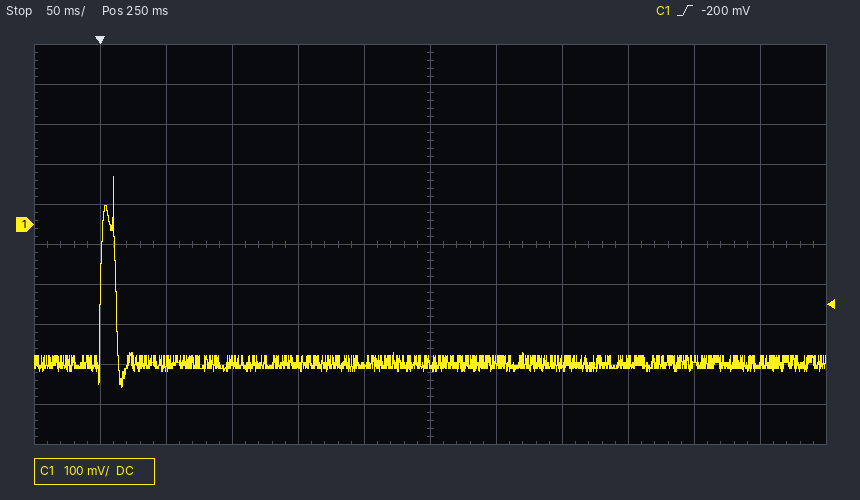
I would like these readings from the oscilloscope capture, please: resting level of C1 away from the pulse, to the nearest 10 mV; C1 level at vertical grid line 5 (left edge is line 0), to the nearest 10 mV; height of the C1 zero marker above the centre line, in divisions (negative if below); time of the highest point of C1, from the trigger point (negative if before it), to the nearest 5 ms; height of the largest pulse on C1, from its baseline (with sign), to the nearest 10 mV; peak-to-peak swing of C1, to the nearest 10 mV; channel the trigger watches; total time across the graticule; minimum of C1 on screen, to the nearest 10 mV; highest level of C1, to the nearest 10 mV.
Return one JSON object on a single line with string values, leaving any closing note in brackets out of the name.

{"resting level of C1 away from the pulse, to the nearest 10 mV": "-340 mV", "C1 level at vertical grid line 5 (left edge is line 0), to the nearest 10 mV": "-350 mV", "height of the C1 zero marker above the centre line, in divisions": "+0.5 div", "time of the highest point of C1, from the trigger point (negative if before it), to the nearest 5 ms": "+10 ms", "height of the largest pulse on C1, from its baseline (with sign), to the nearest 10 mV": "+460 mV", "peak-to-peak swing of C1, to the nearest 10 mV": "530 mV", "channel the trigger watches": "C1", "total time across the graticule": "600 ms", "minimum of C1 on screen, to the nearest 10 mV": "-410 mV", "highest level of C1, to the nearest 10 mV": "120 mV"}
